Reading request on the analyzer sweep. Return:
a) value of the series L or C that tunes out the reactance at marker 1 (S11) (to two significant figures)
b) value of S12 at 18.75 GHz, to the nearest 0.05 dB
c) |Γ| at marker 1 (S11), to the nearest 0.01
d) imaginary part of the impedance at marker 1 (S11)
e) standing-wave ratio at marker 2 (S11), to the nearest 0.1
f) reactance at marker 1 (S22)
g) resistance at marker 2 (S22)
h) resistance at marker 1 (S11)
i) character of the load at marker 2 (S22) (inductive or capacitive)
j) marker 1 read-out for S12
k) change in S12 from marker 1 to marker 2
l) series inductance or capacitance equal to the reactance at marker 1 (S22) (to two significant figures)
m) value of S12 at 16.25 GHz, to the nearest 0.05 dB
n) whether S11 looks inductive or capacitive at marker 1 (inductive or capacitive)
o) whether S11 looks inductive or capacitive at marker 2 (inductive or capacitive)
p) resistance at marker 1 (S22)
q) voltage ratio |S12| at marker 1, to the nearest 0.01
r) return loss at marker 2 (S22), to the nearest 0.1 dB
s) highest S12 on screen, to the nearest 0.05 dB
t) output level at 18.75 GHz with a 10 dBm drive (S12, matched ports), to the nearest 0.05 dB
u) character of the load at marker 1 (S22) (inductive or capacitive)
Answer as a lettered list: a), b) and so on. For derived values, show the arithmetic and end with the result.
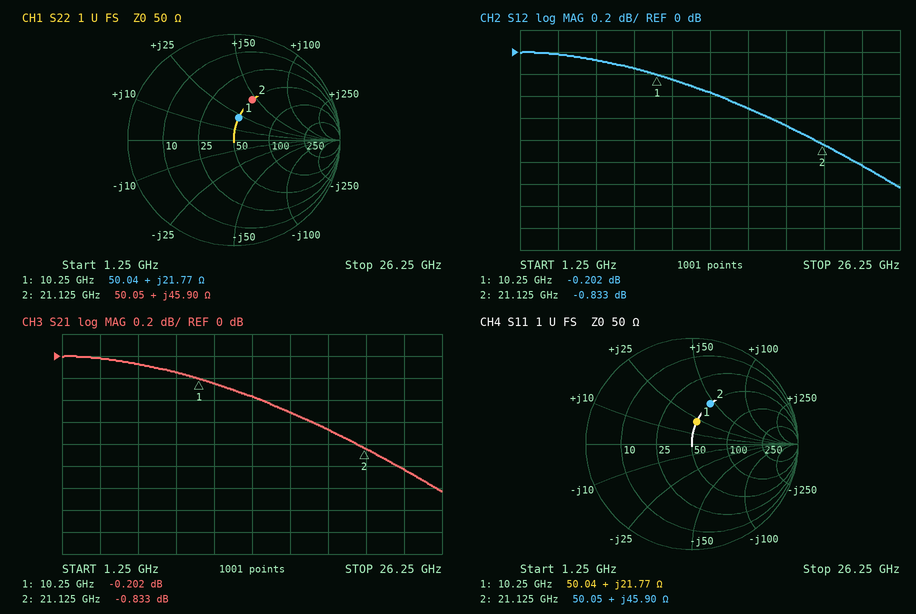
a) C = 1/(2π × 10.25 GHz × 21.77 Ω) ≈ 713 fF, so 710 fF to two significant figures
b) -0.65 dB
c) 0.21
d) +21.77 Ω
e) 2.4
f) +21.77 Ω
g) 50.05 Ω
h) 50.04 Ω
i) inductive
j) -0.202 dB
k) -0.833 − (-0.202) = -0.631 dB
l) L = 21.77 Ω/(2π × 10.25 GHz) ≈ 338 pH, so 340 pH to two significant figures
m) -0.50 dB
n) inductive
o) inductive
p) 50.04 Ω
q) 10^(-0.202/20) ≈ 0.98
r) 7.6 dB
s) 0.00 dB
t) 10 dBm + (-0.65 dB) = 9.35 dBm
u) inductive
